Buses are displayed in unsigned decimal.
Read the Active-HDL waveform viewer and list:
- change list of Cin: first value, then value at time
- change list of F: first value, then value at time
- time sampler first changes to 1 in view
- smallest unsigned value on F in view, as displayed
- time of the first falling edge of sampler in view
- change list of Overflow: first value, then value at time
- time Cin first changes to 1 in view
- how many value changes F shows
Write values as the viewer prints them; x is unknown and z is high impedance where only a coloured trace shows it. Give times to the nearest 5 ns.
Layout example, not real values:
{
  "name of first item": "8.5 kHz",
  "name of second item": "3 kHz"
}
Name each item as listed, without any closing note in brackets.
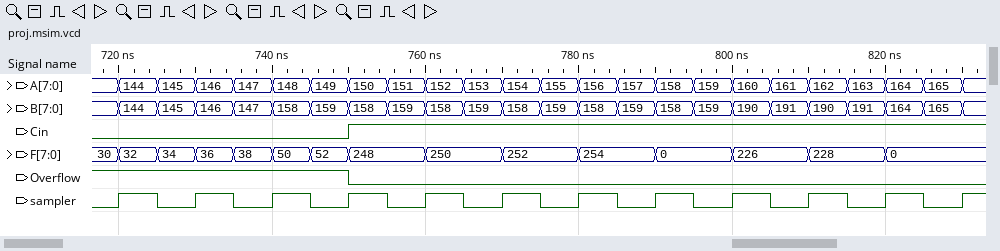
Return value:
{
  "change list of Cin: first value, then value at time": "0, 1 at 750 ns",
  "change list of F: first value, then value at time": "30, 32 at 720 ns, 34 at 725 ns, 36 at 730 ns, 38 at 735 ns, 50 at 740 ns, 52 at 745 ns, 248 at 750 ns, 250 at 760 ns, 252 at 770 ns, 254 at 780 ns, 0 at 790 ns, 226 at 800 ns, 228 at 810 ns, 0 at 820 ns",
  "time sampler first changes to 1 in view": "720 ns",
  "smallest unsigned value on F in view, as displayed": "0",
  "time of the first falling edge of sampler in view": "725 ns",
  "change list of Overflow: first value, then value at time": "1, 0 at 750 ns",
  "time Cin first changes to 1 in view": "750 ns",
  "how many value changes F shows": "14"
}
